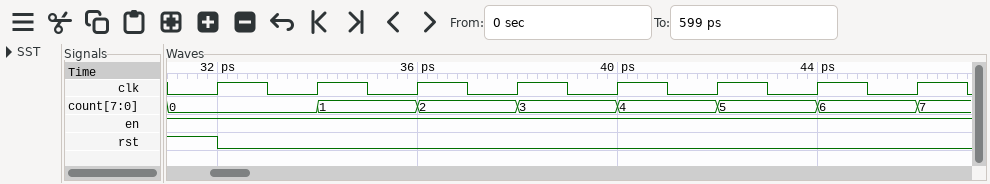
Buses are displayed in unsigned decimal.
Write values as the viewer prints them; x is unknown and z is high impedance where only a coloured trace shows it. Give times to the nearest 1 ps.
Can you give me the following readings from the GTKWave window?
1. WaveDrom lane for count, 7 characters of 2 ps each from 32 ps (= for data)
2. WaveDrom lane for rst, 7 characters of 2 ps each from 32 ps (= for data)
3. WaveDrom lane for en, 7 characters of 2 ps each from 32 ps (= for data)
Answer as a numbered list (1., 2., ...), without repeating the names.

1. {name: 'count', wave: '=======', data: '0 1 2 3 4 5 6'}
2. {name: 'rst', wave: '0......'}
3. {name: 'en', wave: '1......'}
